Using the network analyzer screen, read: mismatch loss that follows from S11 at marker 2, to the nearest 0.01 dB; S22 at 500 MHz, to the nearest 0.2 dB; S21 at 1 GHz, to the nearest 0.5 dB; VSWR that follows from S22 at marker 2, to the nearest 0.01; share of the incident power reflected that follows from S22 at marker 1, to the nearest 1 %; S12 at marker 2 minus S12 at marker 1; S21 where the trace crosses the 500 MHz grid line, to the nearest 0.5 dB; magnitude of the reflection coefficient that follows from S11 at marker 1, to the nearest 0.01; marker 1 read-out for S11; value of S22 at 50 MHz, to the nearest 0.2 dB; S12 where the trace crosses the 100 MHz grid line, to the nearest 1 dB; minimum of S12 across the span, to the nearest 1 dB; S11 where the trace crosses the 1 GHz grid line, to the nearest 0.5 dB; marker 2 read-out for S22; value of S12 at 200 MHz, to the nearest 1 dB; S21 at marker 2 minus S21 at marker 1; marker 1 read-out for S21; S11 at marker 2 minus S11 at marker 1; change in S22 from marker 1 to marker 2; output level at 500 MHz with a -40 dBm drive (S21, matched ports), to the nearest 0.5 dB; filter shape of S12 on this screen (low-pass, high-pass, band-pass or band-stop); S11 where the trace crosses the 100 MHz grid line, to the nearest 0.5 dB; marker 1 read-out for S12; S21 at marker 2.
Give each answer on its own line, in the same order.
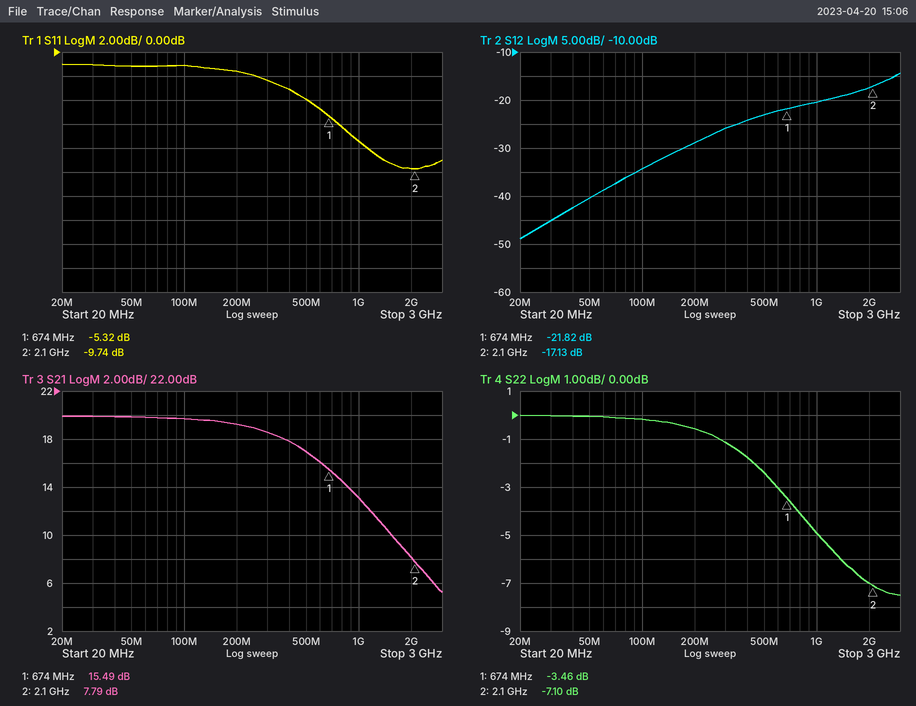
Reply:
0.49 dB
-2.4 dB
13.0 dB
2.58
45 %
4.69 dB
17.0 dB
0.54
-5.32 dB
0.0 dB
-34 dB
-49 dB
-7.5 dB
-7.10 dB
-29 dB
-7.70 dB
15.49 dB
-4.42 dB
-3.64 dB
-23.0 dBm
high-pass
-1.0 dB
-21.82 dB
7.79 dB
